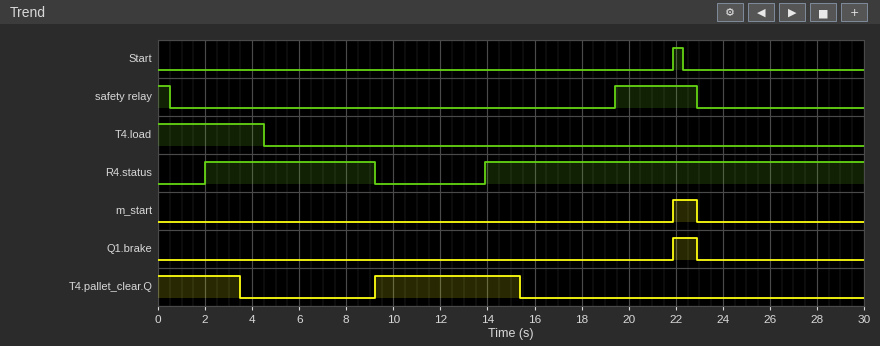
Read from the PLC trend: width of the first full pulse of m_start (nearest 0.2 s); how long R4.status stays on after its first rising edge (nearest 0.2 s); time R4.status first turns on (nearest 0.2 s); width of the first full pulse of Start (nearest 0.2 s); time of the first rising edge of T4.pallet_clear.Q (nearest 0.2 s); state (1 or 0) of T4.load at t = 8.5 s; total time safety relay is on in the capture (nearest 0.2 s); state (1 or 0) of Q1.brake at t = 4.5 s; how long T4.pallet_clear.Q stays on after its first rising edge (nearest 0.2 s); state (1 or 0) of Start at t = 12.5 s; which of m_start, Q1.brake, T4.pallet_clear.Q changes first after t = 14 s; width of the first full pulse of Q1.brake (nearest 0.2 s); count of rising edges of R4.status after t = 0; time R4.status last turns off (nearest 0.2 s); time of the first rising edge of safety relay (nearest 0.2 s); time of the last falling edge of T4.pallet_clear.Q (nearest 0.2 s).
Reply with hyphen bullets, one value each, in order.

- 1.0 s
- 7.2 s
- 2.0 s
- 0.4 s
- 9.2 s
- 0
- 4.0 s
- 0
- 6.2 s
- 0
- T4.pallet_clear.Q
- 1.0 s
- 2
- 9.2 s
- 19.4 s
- 15.4 s
